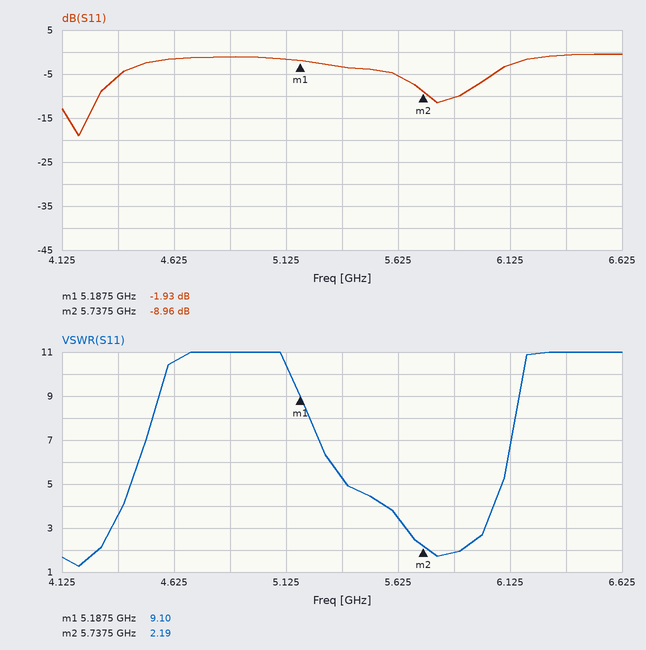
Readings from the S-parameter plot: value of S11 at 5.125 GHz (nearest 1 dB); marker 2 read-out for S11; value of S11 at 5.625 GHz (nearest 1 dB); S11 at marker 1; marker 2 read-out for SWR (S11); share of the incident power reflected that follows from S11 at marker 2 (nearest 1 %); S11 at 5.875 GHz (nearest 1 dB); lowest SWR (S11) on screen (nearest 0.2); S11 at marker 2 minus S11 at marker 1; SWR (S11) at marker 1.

-2 dB
-8.96 dB
-5 dB
-1.93 dB
2.19
13 %
-10 dB
1.2
-7.03 dB
9.10
